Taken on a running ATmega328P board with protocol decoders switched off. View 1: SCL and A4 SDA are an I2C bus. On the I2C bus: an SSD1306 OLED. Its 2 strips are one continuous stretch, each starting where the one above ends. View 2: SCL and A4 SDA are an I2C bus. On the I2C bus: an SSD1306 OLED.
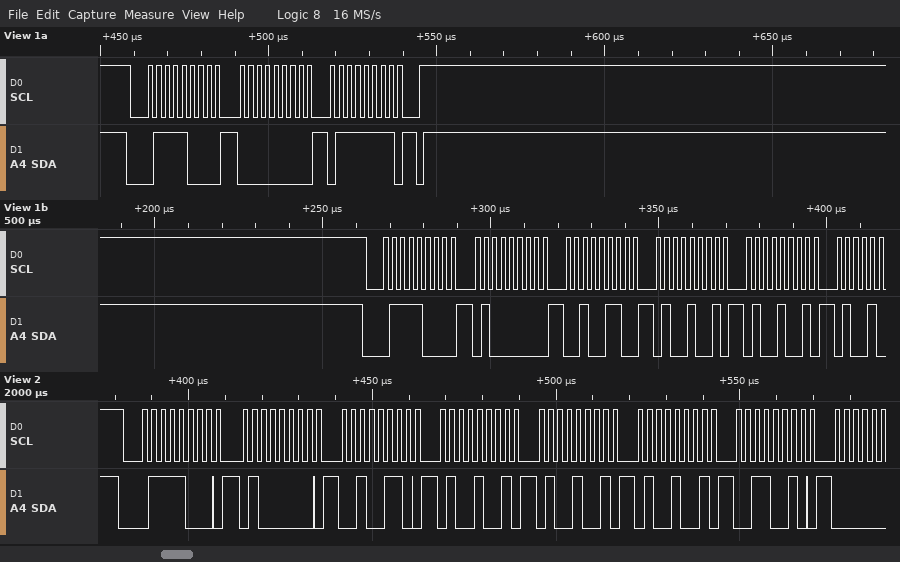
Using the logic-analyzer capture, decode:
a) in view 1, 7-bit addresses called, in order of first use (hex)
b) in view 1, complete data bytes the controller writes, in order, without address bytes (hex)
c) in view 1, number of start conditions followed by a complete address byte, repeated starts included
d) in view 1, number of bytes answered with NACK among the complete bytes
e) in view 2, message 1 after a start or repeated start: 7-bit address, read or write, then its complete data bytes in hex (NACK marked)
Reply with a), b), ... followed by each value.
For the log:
a) 0x3C
b) 00 7F 40 26 49 49
c) 2
d) 0
e) 0x3C write: 40 26 49 49 49 32
